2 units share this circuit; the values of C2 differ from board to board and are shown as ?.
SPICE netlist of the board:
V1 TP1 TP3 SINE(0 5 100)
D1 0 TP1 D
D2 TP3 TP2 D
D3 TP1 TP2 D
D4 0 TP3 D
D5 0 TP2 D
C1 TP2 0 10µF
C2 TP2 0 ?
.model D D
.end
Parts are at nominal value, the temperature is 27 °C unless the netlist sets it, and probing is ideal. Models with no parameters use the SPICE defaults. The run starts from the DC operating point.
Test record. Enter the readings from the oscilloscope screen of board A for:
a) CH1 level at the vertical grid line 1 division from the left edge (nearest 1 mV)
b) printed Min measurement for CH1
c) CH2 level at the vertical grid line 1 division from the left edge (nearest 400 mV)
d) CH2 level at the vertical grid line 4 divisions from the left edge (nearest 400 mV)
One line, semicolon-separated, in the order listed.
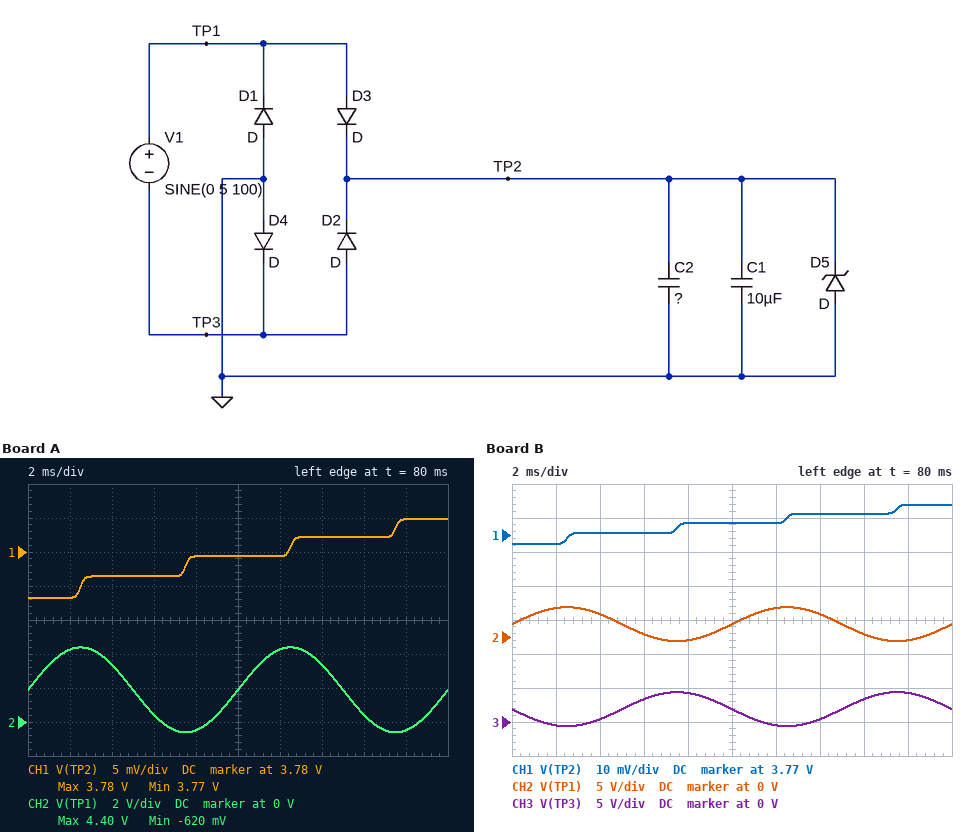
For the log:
3.773 V; 3.77 V; 4.4 V; -400 mV
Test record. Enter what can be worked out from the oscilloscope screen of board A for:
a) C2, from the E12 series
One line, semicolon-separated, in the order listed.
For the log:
15 µF
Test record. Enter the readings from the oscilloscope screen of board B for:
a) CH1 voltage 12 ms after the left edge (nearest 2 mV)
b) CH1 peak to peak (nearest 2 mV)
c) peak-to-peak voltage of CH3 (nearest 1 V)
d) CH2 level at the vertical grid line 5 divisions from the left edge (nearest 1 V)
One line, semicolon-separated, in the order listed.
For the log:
3.774 V; 12 mV; 5 V; 2 V
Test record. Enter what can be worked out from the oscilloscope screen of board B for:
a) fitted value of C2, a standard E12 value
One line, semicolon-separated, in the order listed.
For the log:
18 µF
